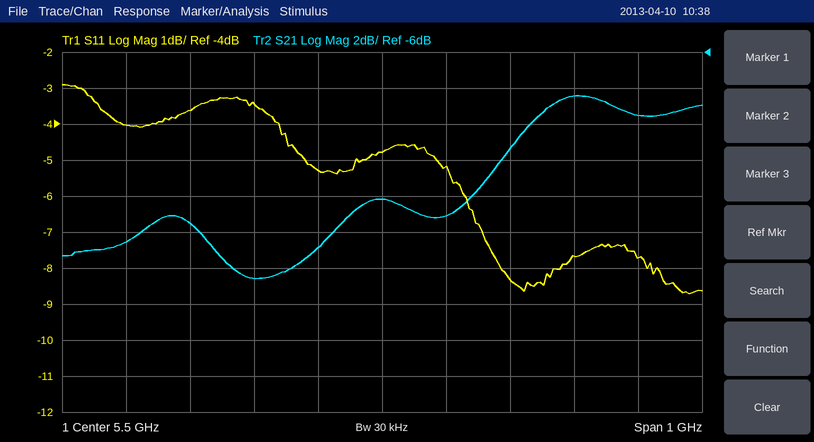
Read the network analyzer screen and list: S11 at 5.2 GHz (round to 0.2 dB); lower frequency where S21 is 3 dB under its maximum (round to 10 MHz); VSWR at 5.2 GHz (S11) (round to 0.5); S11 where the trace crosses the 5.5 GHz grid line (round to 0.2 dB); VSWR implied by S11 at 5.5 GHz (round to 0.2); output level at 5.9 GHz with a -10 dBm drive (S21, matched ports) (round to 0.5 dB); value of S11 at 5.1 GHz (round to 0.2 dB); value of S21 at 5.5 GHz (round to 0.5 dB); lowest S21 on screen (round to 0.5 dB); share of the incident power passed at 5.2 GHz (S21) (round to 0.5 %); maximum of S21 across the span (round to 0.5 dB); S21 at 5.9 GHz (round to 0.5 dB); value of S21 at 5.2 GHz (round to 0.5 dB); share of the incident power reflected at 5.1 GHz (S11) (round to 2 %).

-3.6 dB
5.70 GHz
5.0
-4.8 dB
3.8
-19.5 dBm
-4.0 dB
-14.0 dB
-18.5 dB
3.0 %
-8.5 dB
-9.5 dB
-15.5 dB
40 %
